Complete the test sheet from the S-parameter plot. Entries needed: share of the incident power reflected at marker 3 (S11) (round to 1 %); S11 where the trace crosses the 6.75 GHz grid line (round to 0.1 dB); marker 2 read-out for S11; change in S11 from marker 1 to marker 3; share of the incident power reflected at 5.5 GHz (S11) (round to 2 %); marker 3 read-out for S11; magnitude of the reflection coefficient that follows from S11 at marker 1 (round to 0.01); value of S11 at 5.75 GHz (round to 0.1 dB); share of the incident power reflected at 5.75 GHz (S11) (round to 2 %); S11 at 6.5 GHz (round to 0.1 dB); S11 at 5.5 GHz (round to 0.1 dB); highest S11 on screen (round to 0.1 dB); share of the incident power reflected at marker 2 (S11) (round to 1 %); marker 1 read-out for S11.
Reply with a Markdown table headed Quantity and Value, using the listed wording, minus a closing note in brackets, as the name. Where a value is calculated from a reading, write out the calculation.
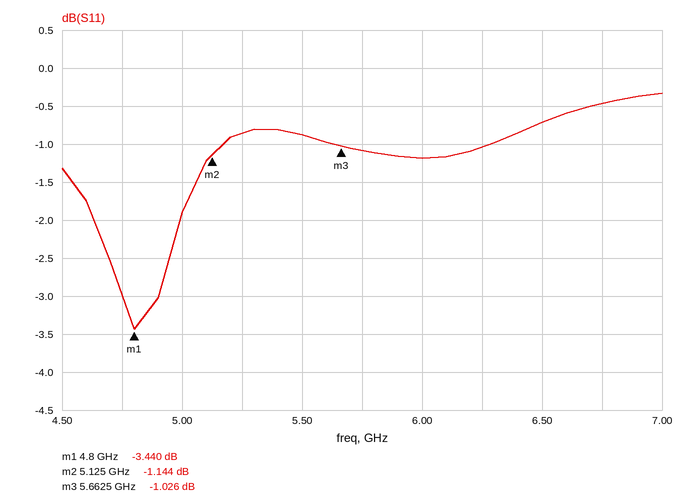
| Quantity | Value |
|---|---|
| share of the incident power reflected at marker 3 (S11) | 10^(-1.026/10) ≈ 79 % |
| S11 where the trace crosses the 6.75 GHz grid line | -0.5 dB |
| marker 2 read-out for S11 | -1.144 dB |
| change in S11 from marker 1 to marker 3 | -1.026 − (-3.44) = 2.414 dB |
| share of the incident power reflected at 5.5 GHz (S11) | 10^(-0.9/10) ≈ 81.3 %, so 82 % to the nearest 2 % |
| marker 3 read-out for S11 | -1.026 dB |
| magnitude of the reflection coefficient that follows from S11 at marker 1 | 10^(-3.44/20) ≈ 0.67 |
| value of S11 at 5.75 GHz | -1.1 dB |
| share of the incident power reflected at 5.75 GHz (S11) | 10^(-1.1/10) ≈ 78 % |
| S11 at 6.5 GHz | -0.7 dB |
| S11 at 5.5 GHz | -0.9 dB |
| highest S11 on screen | -0.3 dB |
| share of the incident power reflected at marker 2 (S11) | 10^(-1.144/10) ≈ 77 % |
| marker 1 read-out for S11 | -3.440 dB |
